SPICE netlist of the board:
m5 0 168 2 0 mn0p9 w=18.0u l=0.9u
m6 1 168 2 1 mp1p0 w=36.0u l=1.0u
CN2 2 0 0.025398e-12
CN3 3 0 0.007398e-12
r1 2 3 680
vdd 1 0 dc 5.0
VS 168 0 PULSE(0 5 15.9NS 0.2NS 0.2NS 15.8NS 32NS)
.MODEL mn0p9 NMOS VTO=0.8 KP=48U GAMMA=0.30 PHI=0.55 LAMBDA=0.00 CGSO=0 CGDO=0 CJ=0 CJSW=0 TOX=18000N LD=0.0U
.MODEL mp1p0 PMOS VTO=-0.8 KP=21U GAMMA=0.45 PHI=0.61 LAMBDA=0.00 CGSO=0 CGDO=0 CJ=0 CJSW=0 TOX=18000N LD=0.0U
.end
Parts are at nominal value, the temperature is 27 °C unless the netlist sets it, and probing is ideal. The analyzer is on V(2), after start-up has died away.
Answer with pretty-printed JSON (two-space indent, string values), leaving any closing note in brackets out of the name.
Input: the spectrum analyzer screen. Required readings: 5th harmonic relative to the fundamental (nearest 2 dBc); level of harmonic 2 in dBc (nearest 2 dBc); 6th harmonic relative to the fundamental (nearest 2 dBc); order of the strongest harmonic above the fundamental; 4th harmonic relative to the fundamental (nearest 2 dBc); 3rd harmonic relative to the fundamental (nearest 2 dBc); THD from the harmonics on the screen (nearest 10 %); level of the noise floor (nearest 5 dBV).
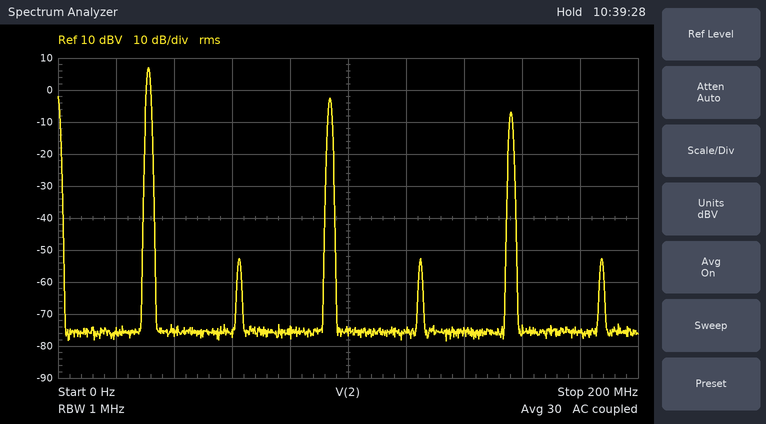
{
  "5th harmonic relative to the fundamental": "-14 dBc",
  "level of harmonic 2 in dBc": "-60 dBc",
  "6th harmonic relative to the fundamental": "-60 dBc",
  "order of the strongest harmonic above the fundamental": "3",
  "4th harmonic relative to the fundamental": "-60 dBc",
  "3rd harmonic relative to the fundamental": "-10 dBc",
  "THD from the harmonics on the screen": "40 %",
  "level of the noise floor": "-75 dBV"
}
